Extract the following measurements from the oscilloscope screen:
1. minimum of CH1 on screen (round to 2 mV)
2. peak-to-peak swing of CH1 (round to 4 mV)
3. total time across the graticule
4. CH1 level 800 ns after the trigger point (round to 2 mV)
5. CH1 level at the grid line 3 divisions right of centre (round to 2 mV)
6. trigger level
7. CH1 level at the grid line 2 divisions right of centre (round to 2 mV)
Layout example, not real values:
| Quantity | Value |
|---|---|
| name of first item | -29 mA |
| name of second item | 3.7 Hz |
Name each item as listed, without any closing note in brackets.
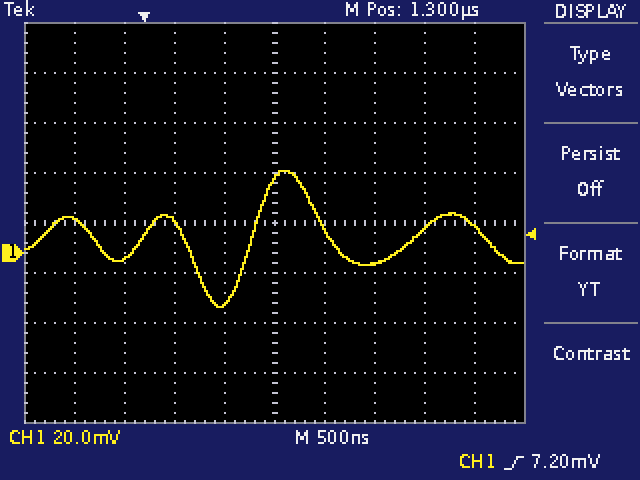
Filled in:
| Quantity | Value |
|---|---|
| minimum of CH1 on screen | -22 mV |
| peak-to-peak swing of CH1 | 56 mV |
| total time across the graticule | 5 µs |
| CH1 level 800 ns after the trigger point | -20 mV |
| CH1 level at the grid line 3 divisions right of centre | 10 mV |
| trigger level | 7.20 mV |
| CH1 level at the grid line 2 divisions right of centre | -4 mV |
